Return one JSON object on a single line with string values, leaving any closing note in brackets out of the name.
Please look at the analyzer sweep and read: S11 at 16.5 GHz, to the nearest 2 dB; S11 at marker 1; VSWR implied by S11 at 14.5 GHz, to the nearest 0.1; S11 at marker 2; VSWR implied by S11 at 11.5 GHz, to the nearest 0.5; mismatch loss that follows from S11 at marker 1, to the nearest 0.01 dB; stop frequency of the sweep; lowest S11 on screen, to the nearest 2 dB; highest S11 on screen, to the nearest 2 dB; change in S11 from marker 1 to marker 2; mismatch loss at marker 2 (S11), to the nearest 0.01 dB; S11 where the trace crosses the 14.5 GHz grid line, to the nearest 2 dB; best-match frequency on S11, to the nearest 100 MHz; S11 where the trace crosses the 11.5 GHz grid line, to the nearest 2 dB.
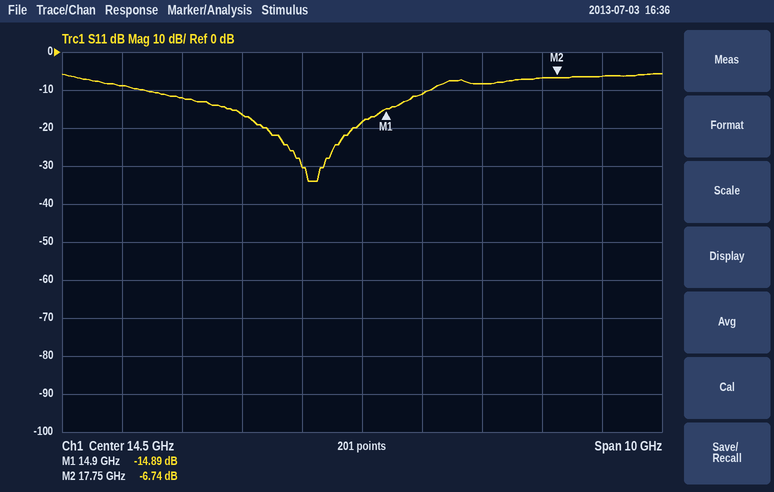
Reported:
{"S11 at 16.5 GHz, to the nearest 2 dB": "-8 dB", "S11 at marker 1": "-14.89 dB", "VSWR implied by S11 at 14.5 GHz, to the nearest 0.1": "1.3", "S11 at marker 2": "-6.74 dB", "VSWR implied by S11 at 11.5 GHz, to the nearest 0.5": "1.5", "mismatch loss that follows from S11 at marker 1, to the nearest 0.01 dB": "0.14 dB", "stop frequency of the sweep": "19.5 GHz", "lowest S11 on screen, to the nearest 2 dB": "-34 dB", "highest S11 on screen, to the nearest 2 dB": "-6 dB", "change in S11 from marker 1 to marker 2": "8.15 dB", "mismatch loss at marker 2 (S11), to the nearest 0.01 dB": "1.03 dB", "S11 where the trace crosses the 14.5 GHz grid line, to the nearest 2 dB": "-18 dB", "best-match frequency on S11, to the nearest 100 MHz": "13.6 GHz", "S11 where the trace crosses the 11.5 GHz grid line, to the nearest 2 dB": "-12 dB"}
